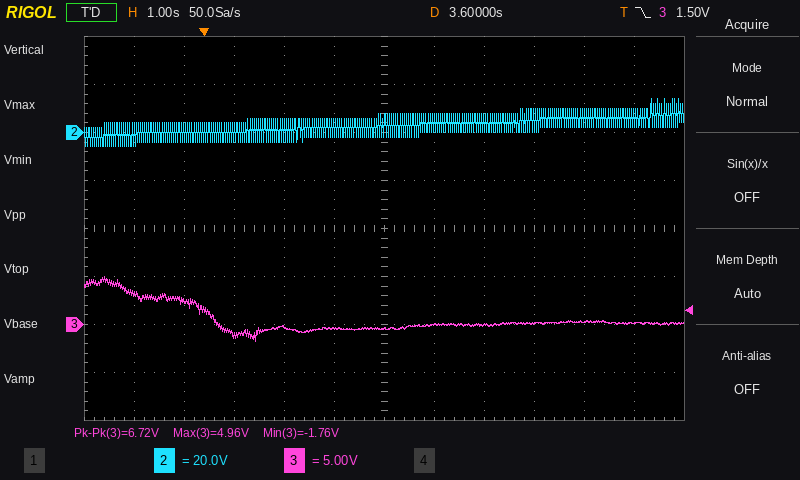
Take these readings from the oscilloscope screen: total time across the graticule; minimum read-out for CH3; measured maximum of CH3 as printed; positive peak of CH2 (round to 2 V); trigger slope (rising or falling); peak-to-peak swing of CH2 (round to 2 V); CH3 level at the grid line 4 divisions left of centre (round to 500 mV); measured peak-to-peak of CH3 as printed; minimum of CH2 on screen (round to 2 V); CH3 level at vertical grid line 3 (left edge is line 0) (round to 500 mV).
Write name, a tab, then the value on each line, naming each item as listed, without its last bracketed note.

total time across the graticule	12 s
minimum read-out for CH3	-1.76 V
measured maximum of CH3 as printed	4.96 V
positive peak of CH2	14 V
trigger slope	falling
peak-to-peak swing of CH2	20 V
CH3 level at the grid line 4 divisions left of centre	2.5 V
measured peak-to-peak of CH3 as printed	6.72 V
minimum of CH2 on screen	-6 V
CH3 level at vertical grid line 3 (left edge is line 0)	-1.0 V
